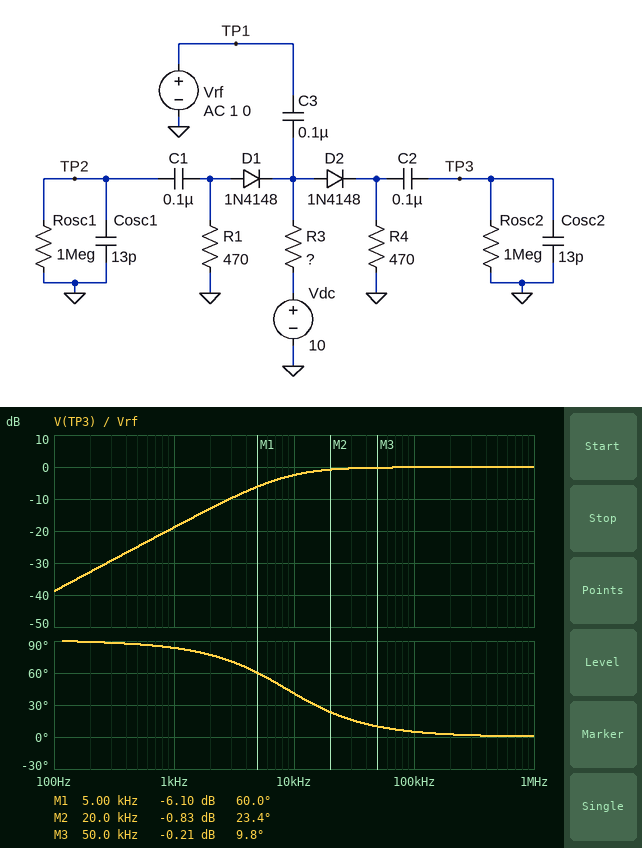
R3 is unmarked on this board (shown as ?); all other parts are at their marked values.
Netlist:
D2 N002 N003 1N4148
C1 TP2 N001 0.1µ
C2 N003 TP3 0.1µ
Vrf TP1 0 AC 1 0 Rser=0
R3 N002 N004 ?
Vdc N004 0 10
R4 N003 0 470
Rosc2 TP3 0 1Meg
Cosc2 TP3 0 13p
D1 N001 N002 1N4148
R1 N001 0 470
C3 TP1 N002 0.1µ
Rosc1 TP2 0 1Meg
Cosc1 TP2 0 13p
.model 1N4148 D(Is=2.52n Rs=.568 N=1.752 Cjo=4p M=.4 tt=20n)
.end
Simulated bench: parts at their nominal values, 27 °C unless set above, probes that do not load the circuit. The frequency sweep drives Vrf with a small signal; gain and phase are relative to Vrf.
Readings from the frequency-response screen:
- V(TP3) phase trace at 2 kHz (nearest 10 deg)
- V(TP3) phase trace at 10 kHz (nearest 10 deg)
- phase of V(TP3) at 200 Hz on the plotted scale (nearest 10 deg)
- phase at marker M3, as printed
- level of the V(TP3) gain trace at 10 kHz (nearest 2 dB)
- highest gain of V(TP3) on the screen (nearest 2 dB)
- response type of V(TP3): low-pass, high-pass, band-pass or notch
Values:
80 deg
40 deg
90 deg
9.8 deg
-2 dB
0 dB
high-pass
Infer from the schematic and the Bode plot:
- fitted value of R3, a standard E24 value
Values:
300 Ω
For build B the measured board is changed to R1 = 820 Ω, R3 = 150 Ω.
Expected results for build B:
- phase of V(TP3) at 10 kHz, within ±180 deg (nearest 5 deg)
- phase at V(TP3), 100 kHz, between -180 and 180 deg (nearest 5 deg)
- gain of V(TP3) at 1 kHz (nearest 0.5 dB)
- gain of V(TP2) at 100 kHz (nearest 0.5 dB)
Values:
55 deg
10 deg
-23.0 dB
-61.5 dB
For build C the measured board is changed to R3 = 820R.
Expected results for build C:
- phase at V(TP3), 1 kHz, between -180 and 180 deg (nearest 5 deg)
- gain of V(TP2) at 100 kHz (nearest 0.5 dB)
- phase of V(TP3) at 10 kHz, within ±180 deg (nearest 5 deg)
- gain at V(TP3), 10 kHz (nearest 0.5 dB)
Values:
80 deg
-64.0 dB
30 deg
-1.0 dB
